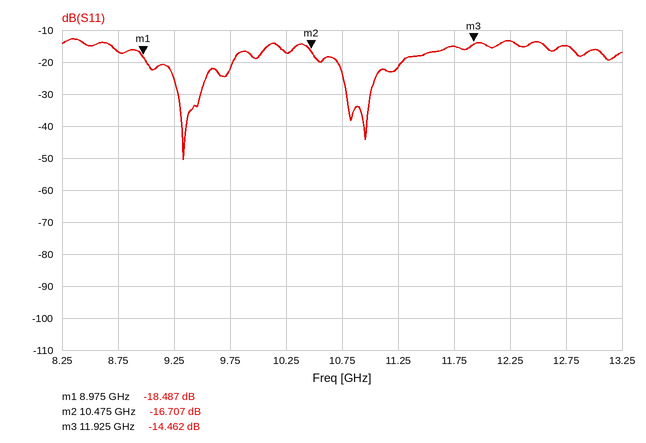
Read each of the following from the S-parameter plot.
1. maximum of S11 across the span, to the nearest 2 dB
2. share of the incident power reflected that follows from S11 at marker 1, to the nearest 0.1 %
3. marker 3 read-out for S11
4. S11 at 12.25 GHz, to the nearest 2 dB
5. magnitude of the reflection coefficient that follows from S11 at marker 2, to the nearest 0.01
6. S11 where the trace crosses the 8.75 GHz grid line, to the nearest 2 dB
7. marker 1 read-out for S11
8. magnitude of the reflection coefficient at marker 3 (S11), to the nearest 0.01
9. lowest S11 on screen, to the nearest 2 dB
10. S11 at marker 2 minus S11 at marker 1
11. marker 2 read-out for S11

-12 dB
1.4 %
-14.462 dB
-14 dB
0.15
-16 dB
-18.487 dB
0.19
-50 dB
1.780 dB
-16.707 dB
